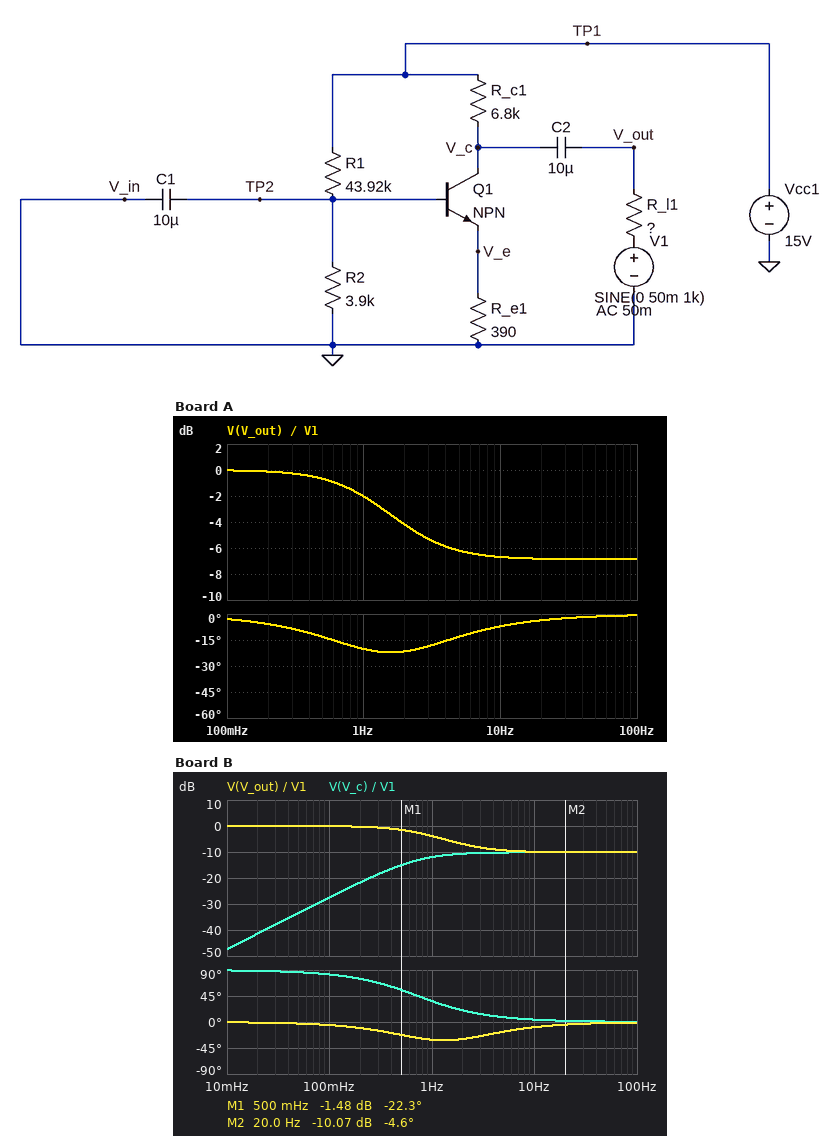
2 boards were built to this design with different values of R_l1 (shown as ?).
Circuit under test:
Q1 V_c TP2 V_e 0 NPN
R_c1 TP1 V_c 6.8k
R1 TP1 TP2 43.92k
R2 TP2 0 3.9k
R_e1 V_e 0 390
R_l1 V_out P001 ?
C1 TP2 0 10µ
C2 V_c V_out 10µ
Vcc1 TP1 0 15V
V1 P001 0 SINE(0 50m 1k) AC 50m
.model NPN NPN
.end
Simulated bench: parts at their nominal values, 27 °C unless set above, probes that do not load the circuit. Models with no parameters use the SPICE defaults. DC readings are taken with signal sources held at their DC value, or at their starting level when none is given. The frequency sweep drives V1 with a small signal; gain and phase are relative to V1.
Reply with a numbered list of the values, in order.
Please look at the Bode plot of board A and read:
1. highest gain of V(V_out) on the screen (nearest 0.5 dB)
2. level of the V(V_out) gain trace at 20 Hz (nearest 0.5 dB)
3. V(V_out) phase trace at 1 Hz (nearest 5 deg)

1. 0 dB
2. -7.0 dB
3. -20 deg
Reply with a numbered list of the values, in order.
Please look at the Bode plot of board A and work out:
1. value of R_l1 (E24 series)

1. 8.2 kΩ
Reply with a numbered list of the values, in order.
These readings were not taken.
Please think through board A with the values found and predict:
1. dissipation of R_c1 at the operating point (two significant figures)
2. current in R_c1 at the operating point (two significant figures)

1. 7.4 mW
2. 1.0 mA
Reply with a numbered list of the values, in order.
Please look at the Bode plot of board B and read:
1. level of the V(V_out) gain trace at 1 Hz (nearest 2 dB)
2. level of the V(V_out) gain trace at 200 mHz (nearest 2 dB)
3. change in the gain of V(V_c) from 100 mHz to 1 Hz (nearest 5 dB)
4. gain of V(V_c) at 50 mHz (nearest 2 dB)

1. -4 dB
2. 0 dB
3. 15 dB
4. -34 dB
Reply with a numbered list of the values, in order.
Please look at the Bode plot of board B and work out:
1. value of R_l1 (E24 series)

1. 15 kΩ
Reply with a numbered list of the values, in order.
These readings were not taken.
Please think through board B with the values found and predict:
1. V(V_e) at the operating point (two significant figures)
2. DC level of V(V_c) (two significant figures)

1. 410 mV
2. 7.9 V
